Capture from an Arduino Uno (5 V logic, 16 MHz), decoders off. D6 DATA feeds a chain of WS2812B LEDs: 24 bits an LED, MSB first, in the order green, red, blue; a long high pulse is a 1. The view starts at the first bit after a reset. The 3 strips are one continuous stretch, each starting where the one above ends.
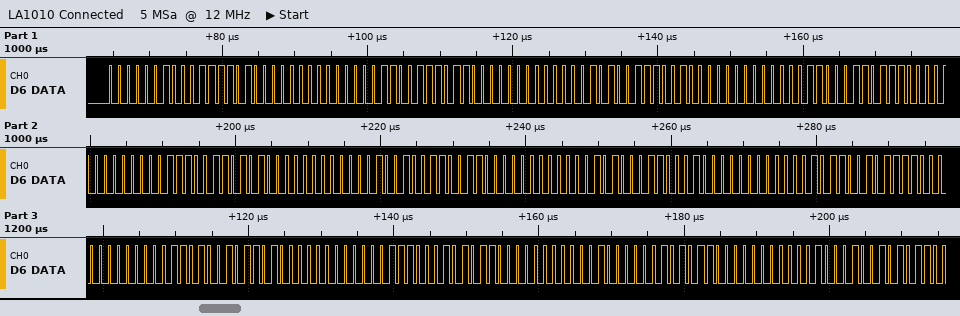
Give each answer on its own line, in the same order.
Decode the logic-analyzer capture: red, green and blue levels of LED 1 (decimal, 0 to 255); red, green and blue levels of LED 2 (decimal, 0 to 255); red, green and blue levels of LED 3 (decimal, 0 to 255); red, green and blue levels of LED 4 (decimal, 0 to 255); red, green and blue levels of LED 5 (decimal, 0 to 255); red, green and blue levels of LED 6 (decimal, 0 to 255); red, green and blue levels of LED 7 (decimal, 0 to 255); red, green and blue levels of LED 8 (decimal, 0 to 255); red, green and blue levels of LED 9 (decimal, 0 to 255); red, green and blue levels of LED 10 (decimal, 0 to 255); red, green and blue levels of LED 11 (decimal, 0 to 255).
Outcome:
61, 2, 0
59, 3, 0
57, 5, 0
55, 6, 0
53, 7, 0
51, 9, 0
49, 10, 0
47, 11, 0
45, 13, 0
43, 14, 0
43, 16, 0
